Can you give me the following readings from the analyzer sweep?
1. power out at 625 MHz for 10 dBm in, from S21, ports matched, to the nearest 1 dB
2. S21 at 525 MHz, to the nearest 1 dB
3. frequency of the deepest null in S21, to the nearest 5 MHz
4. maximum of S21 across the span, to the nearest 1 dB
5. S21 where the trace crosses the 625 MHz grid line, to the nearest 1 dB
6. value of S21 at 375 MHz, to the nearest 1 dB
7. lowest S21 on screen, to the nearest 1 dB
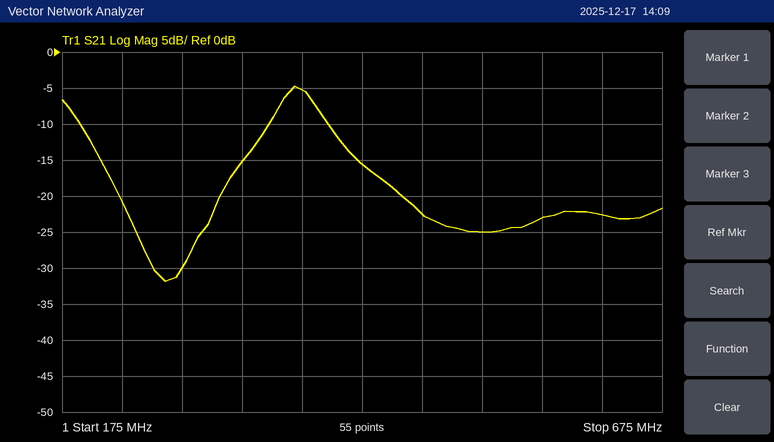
-13 dBm
-25 dB
260 MHz
-5 dB
-23 dB
-5 dB
-32 dB
